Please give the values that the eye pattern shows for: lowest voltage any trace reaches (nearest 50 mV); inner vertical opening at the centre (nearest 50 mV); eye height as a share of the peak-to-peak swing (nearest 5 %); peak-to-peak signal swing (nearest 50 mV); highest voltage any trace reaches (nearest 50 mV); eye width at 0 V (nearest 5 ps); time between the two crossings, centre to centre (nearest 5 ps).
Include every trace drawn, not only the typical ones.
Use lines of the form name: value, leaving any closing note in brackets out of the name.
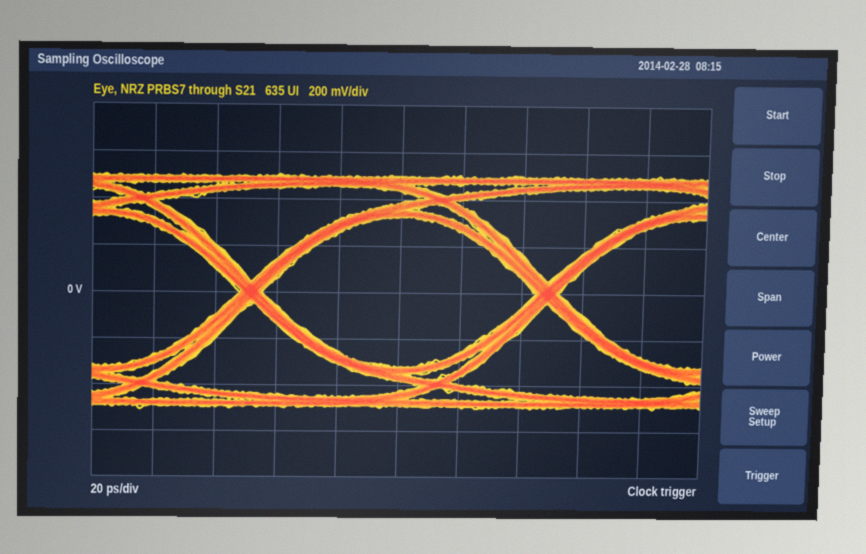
lowest voltage any trace reaches: -500 mV
inner vertical opening at the centre: 650 mV
eye height as a share of the peak-to-peak swing: 65 %
peak-to-peak signal swing: 1.00 V
highest voltage any trace reaches: 500 mV
eye width at 0 V: 90 ps
time between the two crossings, centre to centre: 95 ps
